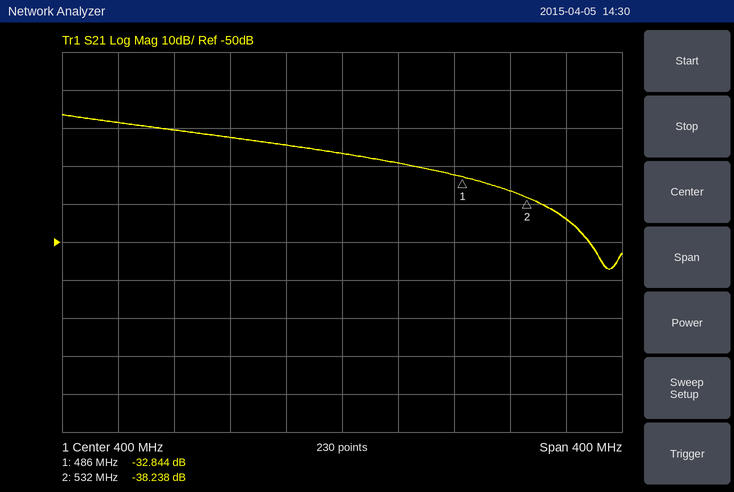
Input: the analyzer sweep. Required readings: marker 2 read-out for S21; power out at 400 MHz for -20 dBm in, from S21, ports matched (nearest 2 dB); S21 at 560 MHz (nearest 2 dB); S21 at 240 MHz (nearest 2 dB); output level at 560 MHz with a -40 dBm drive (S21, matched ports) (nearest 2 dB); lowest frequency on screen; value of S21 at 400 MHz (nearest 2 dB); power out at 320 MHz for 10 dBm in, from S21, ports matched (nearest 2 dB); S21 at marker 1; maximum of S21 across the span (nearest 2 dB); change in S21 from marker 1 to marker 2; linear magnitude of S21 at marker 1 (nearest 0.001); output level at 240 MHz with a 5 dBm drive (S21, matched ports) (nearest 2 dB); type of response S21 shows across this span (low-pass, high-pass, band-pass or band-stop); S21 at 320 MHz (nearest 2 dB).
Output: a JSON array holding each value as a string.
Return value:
["-38.238 dB", "-46 dBm", "-44 dB", "-18 dB", "-84 dBm", "200 MHz", "-26 dB", "-12 dBm", "-32.844 dB", "-16 dB", "-5.394 dB", "0.023", "-14 dBm", "low-pass", "-22 dB"]
